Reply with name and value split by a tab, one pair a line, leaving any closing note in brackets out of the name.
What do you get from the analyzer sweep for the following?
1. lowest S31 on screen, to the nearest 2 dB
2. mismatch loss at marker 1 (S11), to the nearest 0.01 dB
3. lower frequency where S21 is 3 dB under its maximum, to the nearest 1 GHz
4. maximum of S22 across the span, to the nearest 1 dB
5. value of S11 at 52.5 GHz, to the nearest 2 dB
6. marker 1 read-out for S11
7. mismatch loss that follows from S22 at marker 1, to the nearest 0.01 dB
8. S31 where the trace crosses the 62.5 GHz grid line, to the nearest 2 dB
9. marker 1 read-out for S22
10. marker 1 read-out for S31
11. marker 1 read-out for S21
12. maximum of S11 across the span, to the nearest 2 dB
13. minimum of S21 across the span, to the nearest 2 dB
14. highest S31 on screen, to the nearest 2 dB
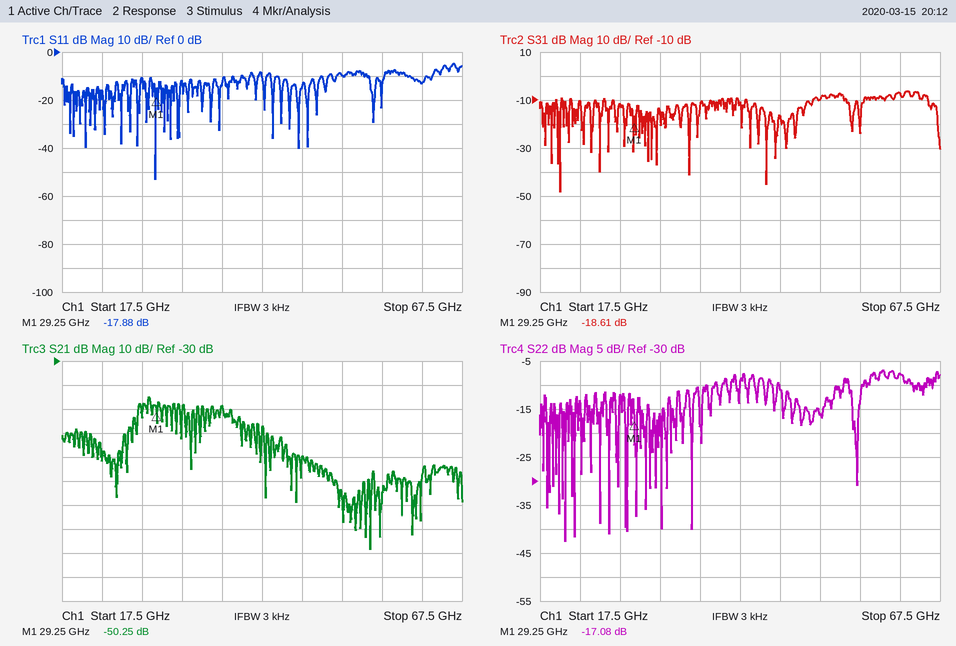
lowest S31 on screen, to the nearest 2 dB	-48 dB
mismatch loss at marker 1 (S11), to the nearest 0.01 dB	0.07 dB
lower frequency where S21 is 3 dB under its maximum, to the nearest 1 GHz	28 GHz
maximum of S22 across the span, to the nearest 1 dB	-7 dB
value of S11 at 52.5 GHz, to the nearest 2 dB	-10 dB
marker 1 read-out for S11	-17.88 dB
mismatch loss that follows from S22 at marker 1, to the nearest 0.01 dB	0.09 dB
S31 where the trace crosses the 62.5 GHz grid line, to the nearest 2 dB	-8 dB
marker 1 read-out for S22	-17.08 dB
marker 1 read-out for S31	-18.61 dB
marker 1 read-out for S21	-50.25 dB
maximum of S11 across the span, to the nearest 2 dB	-4 dB
minimum of S21 across the span, to the nearest 2 dB	-108 dB
highest S31 on screen, to the nearest 2 dB	-6 dB
